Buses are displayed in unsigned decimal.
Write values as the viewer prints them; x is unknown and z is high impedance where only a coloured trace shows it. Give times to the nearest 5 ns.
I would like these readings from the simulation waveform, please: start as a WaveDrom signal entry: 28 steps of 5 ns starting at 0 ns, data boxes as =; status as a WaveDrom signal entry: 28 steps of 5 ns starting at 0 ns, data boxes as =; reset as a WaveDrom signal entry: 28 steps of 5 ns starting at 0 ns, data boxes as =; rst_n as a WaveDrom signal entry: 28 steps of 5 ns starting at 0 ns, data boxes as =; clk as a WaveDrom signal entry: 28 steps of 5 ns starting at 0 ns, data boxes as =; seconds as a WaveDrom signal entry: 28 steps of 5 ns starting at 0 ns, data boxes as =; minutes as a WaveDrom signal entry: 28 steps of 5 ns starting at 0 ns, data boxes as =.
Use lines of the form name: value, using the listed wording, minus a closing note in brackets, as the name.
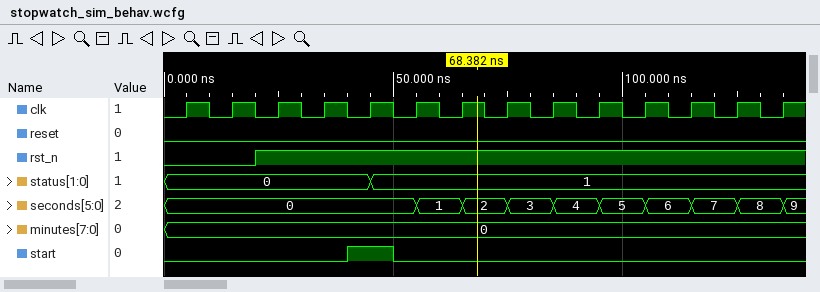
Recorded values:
start as a WaveDrom signal entry: 28 steps of 5 ns starting at 0 ns, data boxes as =: {name: 'start', wave: '0.......1.0.................'}
status as a WaveDrom signal entry: 28 steps of 5 ns starting at 0 ns, data boxes as =: {name: 'status', wave: '=........=..................', data: '0 1'}
reset as a WaveDrom signal entry: 28 steps of 5 ns starting at 0 ns, data boxes as =: {name: 'reset', wave: '0...........................'}
rst_n as a WaveDrom signal entry: 28 steps of 5 ns starting at 0 ns, data boxes as =: {name: 'rst_n', wave: '0...1.......................'}
clk as a WaveDrom signal entry: 28 steps of 5 ns starting at 0 ns, data boxes as =: {name: 'clk', wave: '0101010101010101010101010101'}
seconds as a WaveDrom signal entry: 28 steps of 5 ns starting at 0 ns, data boxes as =: {name: 'seconds', wave: '=..........=.=.=.=.=.=.=.=.=', data: '0 1 2 3 4 5 6 7 8 9'}
minutes as a WaveDrom signal entry: 28 steps of 5 ns starting at 0 ns, data boxes as =: {name: 'minutes', wave: '=...........................', data: '0'}
